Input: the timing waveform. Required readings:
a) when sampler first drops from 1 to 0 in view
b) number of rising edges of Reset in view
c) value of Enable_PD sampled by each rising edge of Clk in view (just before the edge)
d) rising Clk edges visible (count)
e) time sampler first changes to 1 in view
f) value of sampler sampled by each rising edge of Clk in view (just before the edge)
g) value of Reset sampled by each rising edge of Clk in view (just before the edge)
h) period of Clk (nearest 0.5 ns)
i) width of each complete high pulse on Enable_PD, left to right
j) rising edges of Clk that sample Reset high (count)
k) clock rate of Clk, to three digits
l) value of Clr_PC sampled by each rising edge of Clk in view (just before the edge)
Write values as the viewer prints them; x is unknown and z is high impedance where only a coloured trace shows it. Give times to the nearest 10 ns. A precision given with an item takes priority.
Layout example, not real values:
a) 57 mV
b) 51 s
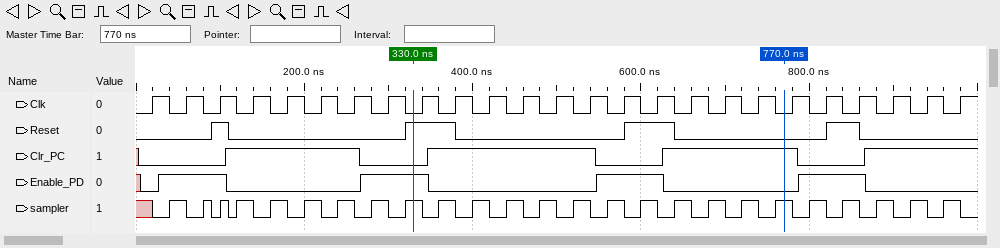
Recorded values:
a) 60 ns
b) 4
c) 0 1 1 0 0 0 0 1 1 0 0 0 0 0 1 1 0 0 0 0 1 1 0 0 0
d) 25
e) 40 ns
f) x 1 0 1 1 1 1 1 1 1 1 1 1 1 1 1 1 1 1 1 1 1 1 1 1
g) 0 0 1 0 0 0 0 0 1 1 0 0 0 0 0 1 0 0 0 0 0 1 0 0 0
h) 40 ns
i) 80 ns, 80 ns, 80 ns, 80 ns
j) 5
k) 25.0 MHz
l) 0 0 0 1 1 1 1 0 0 1 1 1 1 1 0 0 1 1 1 1 0 0 1 1 1
